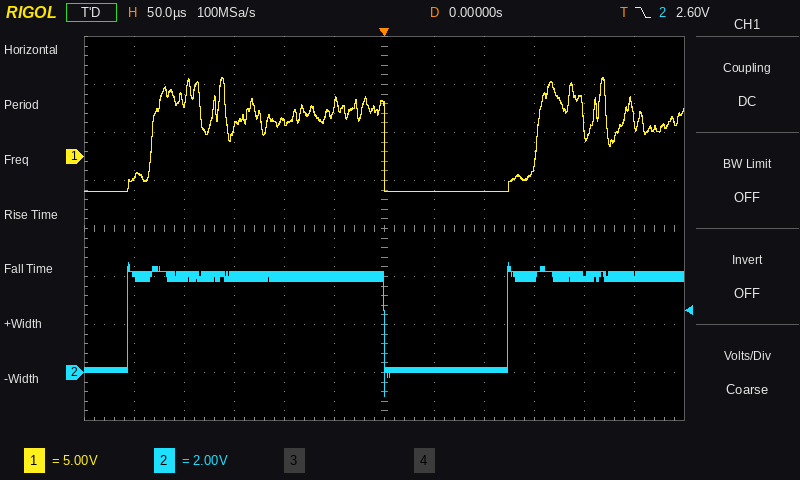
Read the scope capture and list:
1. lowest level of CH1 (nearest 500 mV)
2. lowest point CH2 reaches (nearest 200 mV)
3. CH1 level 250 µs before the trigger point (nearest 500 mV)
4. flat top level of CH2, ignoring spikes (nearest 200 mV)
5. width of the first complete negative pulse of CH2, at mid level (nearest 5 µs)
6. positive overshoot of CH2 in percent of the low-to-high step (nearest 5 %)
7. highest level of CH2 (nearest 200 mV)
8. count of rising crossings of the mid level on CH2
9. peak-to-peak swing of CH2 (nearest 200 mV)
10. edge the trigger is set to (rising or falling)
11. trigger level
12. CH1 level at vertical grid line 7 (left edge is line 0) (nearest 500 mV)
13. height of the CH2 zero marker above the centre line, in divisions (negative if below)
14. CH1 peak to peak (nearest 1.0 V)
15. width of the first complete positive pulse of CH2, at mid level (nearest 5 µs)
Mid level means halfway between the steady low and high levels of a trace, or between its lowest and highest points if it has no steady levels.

-3.5 V
-1.0 V
-2.0 V
4.0 V
125 µs
15 %
4.6 V
2
5.6 V
falling
2.60 V
-3.5 V
-3.0 div
12.0 V
255 µs
